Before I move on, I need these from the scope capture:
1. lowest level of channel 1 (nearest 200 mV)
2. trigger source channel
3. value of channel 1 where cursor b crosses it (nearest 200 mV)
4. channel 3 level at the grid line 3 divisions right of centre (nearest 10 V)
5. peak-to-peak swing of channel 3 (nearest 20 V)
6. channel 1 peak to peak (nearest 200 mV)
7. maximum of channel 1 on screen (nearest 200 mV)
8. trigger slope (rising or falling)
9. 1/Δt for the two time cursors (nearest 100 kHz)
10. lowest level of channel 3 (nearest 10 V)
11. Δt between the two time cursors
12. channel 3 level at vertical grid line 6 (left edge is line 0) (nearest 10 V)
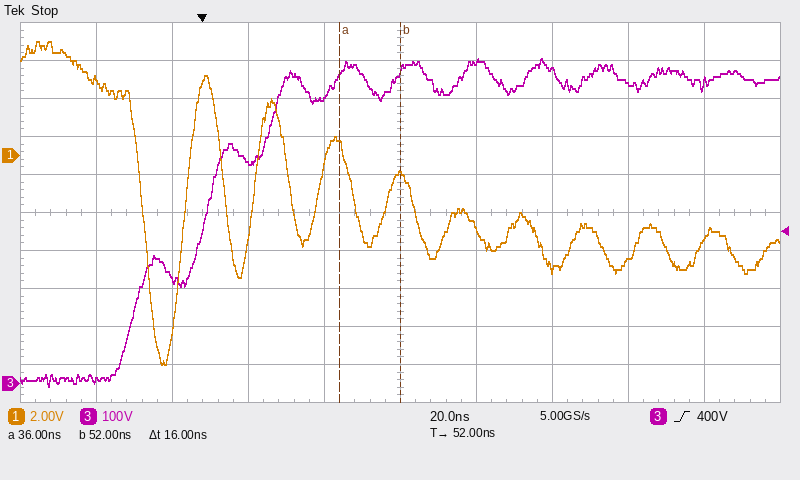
-11.0 V
channel 3
-1.0 V
790 V
860 V
17.0 V
6.0 V
rising
62.5 MHz
-10 V
16 ns
850 V
